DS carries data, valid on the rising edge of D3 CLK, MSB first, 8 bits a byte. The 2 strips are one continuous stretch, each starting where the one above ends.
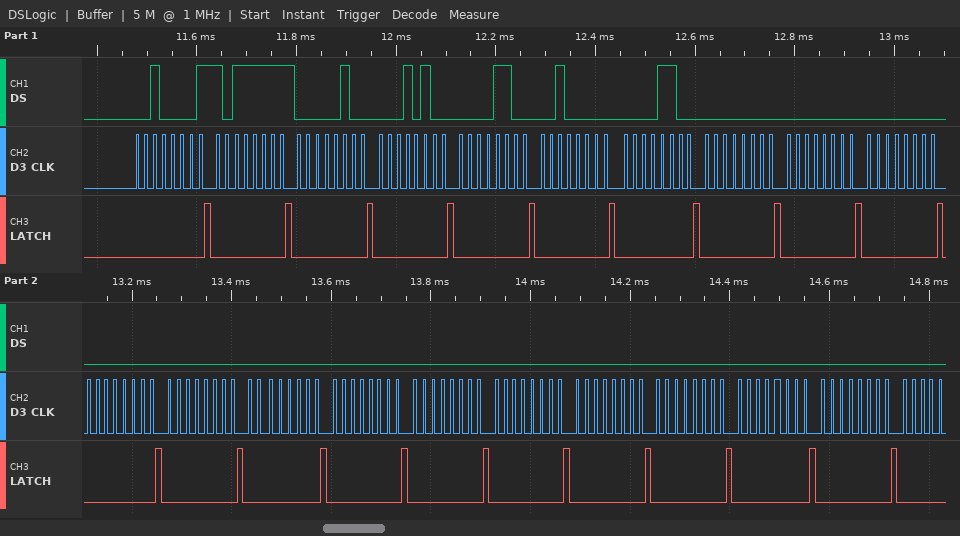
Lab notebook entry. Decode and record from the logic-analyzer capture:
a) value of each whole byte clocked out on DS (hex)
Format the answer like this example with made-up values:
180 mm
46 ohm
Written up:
21 BF 04 14 0C 20 0C 00 00 00 00 00 00 00 00 00 00 00 00 00
